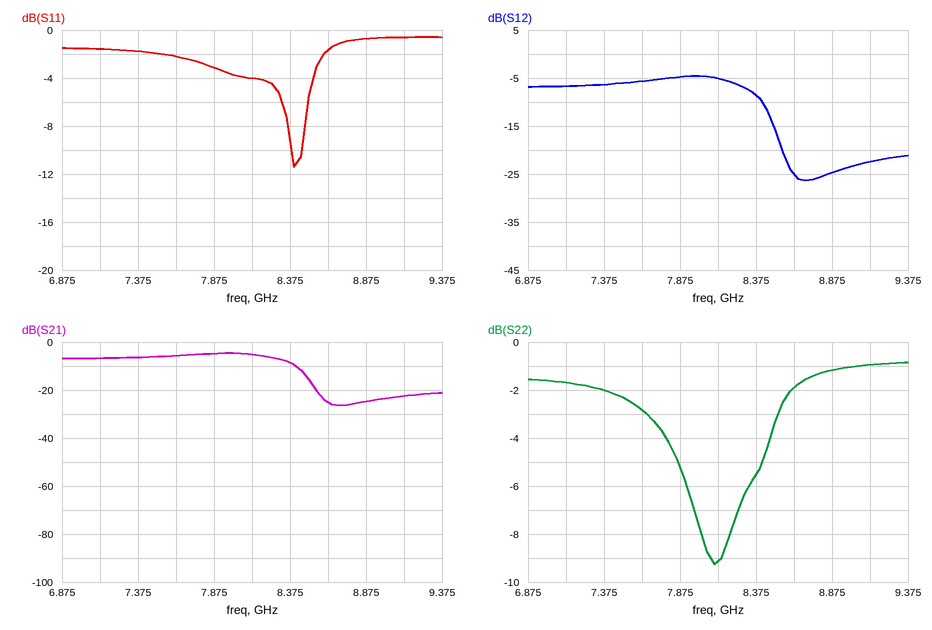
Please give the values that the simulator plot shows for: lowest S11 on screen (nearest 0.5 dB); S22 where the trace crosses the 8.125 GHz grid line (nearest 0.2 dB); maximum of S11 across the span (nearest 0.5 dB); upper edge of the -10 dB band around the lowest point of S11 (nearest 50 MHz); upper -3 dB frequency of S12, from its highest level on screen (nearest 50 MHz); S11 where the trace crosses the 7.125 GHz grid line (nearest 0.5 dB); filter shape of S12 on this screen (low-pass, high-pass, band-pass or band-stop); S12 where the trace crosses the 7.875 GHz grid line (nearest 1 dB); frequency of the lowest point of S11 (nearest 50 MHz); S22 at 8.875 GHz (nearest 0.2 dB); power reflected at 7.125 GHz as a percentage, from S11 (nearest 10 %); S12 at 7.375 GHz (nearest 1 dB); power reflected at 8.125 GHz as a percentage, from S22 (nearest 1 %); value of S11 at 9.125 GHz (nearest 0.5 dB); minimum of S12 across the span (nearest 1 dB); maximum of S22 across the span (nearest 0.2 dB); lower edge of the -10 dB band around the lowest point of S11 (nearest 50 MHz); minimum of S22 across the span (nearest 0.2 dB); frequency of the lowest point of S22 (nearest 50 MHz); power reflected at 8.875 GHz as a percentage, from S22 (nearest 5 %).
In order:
-11.5 dB
-9.2 dB
-0.5 dB
8.45 GHz
8.35 GHz
-1.5 dB
low-pass
-5 dB
8.40 GHz
-1.2 dB
70 %
-6 dB
12 %
-0.5 dB
-26 dB
-0.8 dB
8.40 GHz
-9.2 dB
8.10 GHz
75 %
